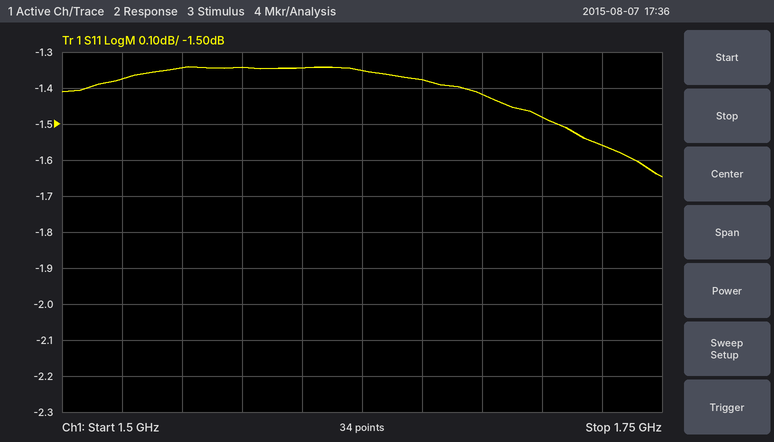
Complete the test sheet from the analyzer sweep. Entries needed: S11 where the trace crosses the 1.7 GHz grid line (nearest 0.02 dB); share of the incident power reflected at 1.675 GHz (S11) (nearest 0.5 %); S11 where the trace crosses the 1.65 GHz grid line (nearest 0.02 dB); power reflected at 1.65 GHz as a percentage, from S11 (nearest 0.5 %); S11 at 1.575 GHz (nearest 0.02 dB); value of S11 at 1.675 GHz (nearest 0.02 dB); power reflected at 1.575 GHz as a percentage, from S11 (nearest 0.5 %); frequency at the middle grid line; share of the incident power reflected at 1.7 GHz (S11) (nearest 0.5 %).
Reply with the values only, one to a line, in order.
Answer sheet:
-1.48 dB
72.0 %
-1.38 dB
73.0 %
-1.34 dB
-1.42 dB
73.5 %
1.625 GHz
71.0 %
